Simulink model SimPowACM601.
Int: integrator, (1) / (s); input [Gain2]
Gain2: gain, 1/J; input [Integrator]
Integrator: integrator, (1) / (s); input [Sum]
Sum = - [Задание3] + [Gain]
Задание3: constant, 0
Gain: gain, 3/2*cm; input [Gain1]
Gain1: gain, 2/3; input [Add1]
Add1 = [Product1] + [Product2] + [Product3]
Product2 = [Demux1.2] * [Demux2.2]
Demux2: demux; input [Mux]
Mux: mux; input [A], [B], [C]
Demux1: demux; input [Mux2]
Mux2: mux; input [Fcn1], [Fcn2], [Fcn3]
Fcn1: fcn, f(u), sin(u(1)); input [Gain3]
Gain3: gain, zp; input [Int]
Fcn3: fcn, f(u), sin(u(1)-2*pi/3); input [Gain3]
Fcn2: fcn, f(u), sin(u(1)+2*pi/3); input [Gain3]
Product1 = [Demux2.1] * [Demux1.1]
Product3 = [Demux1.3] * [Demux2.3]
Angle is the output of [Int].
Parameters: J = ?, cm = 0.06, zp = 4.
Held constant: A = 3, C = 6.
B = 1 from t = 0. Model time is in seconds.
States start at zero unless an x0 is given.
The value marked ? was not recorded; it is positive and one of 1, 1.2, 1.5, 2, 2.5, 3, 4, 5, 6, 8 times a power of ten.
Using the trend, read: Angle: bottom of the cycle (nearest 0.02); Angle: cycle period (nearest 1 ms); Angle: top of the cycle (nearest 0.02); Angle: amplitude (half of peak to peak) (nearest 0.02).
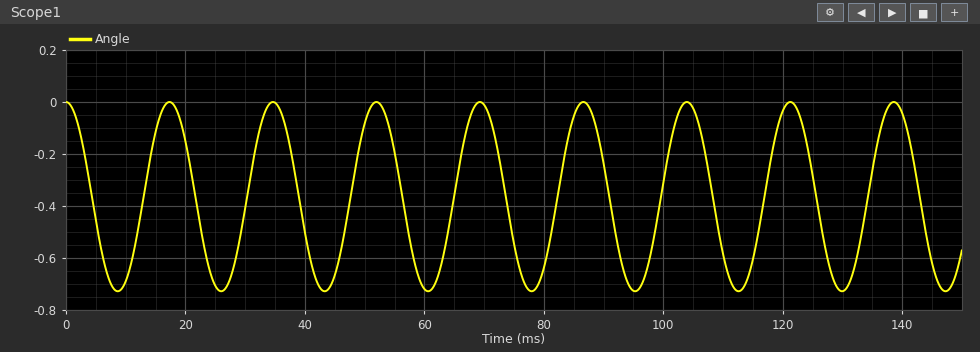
-0.72
17 ms
0.00
0.36
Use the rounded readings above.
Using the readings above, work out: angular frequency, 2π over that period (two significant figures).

0.37 rad/ms
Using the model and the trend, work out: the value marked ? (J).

6e-06
